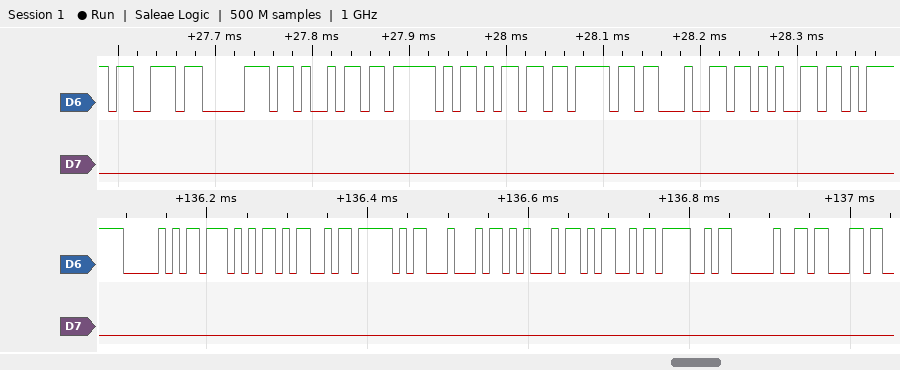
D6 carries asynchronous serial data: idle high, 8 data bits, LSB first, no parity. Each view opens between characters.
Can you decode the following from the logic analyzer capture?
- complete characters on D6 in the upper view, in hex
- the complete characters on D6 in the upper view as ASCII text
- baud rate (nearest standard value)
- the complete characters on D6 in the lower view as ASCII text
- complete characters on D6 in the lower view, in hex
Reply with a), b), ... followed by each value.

a) 73, 70, 69, 5F, 6D, 6F, 64, 65
b) "spi_mode"
c) 115200 baud
d) "PWM_DEMO c"
e) 50, 57, 4D, 5F, 44, 45, 4D, 4F, 20, 63
